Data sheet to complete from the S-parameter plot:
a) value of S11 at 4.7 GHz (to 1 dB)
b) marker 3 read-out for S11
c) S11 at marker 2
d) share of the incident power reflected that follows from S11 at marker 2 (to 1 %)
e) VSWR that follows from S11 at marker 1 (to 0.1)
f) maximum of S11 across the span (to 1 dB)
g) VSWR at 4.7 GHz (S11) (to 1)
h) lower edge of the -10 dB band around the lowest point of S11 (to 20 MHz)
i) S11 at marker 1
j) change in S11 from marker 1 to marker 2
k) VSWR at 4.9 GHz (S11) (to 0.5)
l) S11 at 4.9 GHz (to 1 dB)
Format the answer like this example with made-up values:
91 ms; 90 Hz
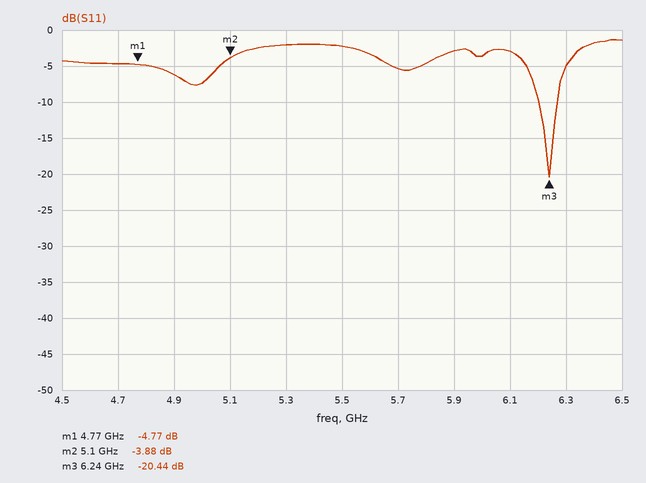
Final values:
-5 dB; -20.44 dB; -3.88 dB; 41 %; 3.7; -1 dB; 4; 6.20 GHz; -4.77 dB; 0.89 dB; 3.0; -6 dB
